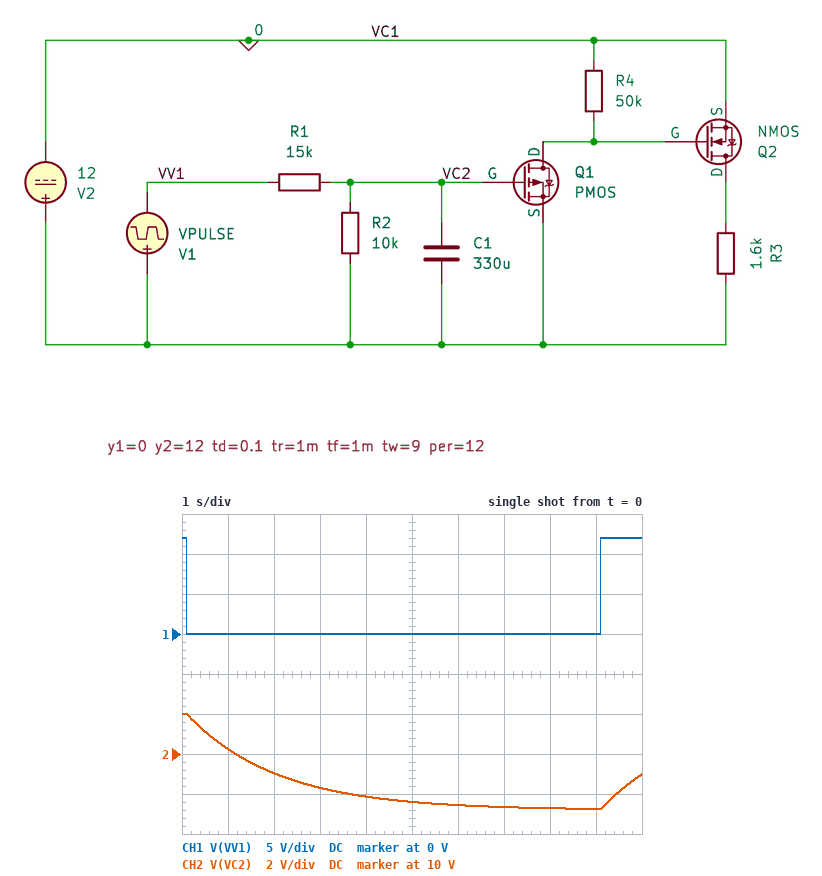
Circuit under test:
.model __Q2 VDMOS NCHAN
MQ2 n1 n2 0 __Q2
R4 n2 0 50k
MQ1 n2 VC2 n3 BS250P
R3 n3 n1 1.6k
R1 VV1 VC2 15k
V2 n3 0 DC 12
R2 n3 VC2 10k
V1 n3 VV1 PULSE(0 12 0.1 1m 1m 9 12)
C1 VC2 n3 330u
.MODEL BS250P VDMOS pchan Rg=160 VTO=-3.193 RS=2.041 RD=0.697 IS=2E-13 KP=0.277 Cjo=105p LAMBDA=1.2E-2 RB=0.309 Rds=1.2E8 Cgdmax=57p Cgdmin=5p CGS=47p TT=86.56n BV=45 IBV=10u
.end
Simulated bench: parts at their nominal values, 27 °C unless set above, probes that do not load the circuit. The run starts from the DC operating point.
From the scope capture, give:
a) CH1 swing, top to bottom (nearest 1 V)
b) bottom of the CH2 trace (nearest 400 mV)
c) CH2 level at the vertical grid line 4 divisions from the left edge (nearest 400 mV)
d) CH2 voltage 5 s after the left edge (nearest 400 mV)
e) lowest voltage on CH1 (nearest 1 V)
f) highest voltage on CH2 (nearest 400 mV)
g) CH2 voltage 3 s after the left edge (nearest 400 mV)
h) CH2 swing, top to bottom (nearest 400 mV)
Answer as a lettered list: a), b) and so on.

a) 12 V
b) 7.2 V
c) 8.0 V
d) 7.6 V
e) 0 V
f) 12.0 V
g) 8.4 V
h) 4.8 V
